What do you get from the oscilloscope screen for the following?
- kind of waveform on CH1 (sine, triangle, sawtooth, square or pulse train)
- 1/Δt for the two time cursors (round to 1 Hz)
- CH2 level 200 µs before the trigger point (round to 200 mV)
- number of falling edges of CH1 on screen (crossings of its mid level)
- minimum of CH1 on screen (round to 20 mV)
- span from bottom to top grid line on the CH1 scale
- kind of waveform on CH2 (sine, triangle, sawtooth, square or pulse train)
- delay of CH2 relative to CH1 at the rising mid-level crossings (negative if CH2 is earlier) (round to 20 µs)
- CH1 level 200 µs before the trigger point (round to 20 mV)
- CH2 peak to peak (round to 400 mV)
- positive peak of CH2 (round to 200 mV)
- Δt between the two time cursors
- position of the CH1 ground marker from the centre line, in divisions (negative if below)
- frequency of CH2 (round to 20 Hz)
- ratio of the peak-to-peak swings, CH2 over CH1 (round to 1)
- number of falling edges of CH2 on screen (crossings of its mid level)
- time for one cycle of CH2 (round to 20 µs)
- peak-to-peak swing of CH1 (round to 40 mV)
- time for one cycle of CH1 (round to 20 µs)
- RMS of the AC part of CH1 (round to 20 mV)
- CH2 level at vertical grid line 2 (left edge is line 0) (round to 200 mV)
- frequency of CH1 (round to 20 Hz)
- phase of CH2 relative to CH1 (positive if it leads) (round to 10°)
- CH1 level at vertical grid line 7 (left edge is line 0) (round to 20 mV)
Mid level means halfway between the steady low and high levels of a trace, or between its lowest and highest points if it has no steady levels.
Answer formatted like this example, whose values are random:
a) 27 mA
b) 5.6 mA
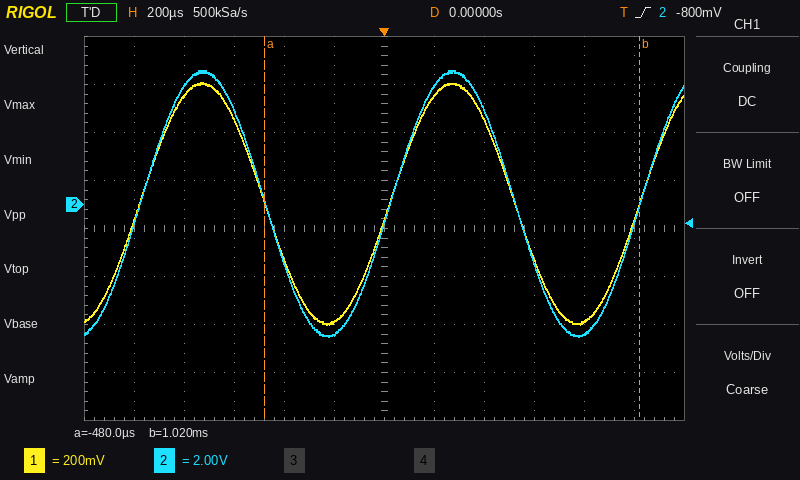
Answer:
a) sine
b) 667 Hz
c) -5.4 V
d) 2
e) -500 mV
f) 1.6 V
g) sine
h) 0 µs
i) -480 mV
j) 11.2 V
k) 5.6 V
l) 1.50 ms
m) +0.5 div
n) 1.00 kHz
o) 11
p) 2
q) 1.00 ms
r) 1.00 V
s) 1.00 ms
t) 360 mV
u) 5.0 V
v) 1.00 kHz
w) 0°
x) 460 mV
